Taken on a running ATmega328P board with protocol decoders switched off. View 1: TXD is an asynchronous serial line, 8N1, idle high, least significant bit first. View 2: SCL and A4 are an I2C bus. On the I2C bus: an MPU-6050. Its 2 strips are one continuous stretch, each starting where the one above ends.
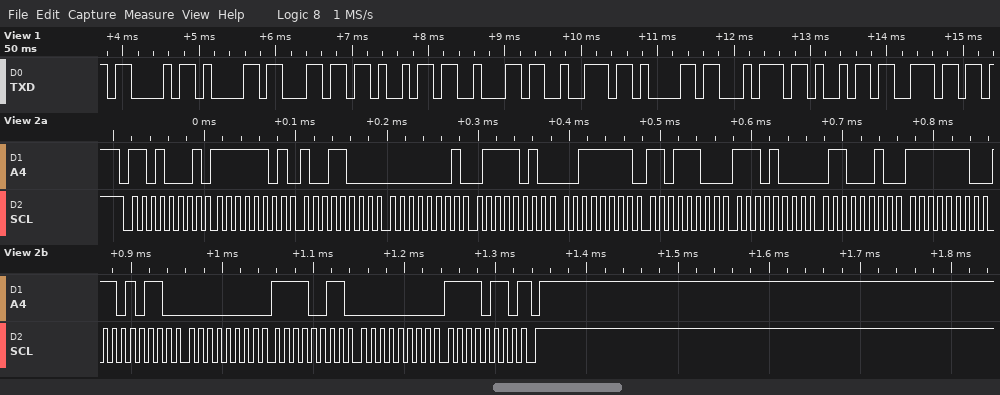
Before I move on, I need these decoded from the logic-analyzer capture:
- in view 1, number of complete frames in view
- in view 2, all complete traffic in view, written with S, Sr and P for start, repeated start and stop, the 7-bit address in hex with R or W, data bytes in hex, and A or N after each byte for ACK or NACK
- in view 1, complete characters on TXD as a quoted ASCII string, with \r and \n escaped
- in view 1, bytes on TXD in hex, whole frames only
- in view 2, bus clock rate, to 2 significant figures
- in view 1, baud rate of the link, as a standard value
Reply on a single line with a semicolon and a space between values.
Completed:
10; S 68R A FD A 98 A 01 A 7A A 3F A DC A E8 A 62 A FE A D6 A 00 A F3 A 00 A F6 N P; "Calibratin"; 0x43 0x61 0x6C 0x69 0x62 0x72 0x61 0x74 0x69 0x6E; 100 kHz; 9600 baud
